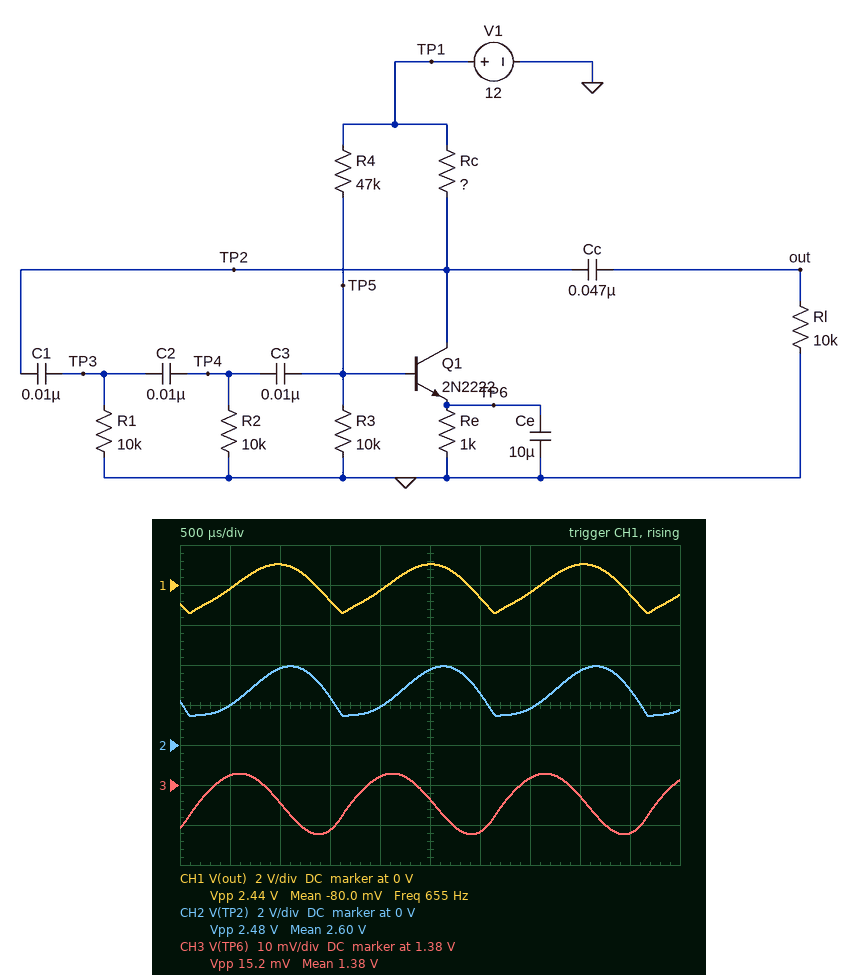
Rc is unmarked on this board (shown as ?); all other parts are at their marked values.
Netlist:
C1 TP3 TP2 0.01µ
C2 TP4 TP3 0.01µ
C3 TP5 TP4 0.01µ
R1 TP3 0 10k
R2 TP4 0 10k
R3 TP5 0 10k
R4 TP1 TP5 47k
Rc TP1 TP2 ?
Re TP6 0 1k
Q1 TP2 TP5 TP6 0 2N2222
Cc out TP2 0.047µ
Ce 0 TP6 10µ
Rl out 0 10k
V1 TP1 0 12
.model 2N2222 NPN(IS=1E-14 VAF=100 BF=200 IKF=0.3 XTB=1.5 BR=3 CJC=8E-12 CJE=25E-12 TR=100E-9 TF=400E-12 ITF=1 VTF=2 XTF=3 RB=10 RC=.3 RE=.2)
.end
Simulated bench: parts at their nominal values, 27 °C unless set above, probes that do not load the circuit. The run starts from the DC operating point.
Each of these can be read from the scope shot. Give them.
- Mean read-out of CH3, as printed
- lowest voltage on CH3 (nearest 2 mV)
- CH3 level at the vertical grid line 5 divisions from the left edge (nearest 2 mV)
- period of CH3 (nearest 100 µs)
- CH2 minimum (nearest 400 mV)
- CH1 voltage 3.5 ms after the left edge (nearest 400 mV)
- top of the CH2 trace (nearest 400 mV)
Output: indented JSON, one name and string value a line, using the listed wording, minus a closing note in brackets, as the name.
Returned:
{
  "Mean read-out of CH3, as printed": "1.38 V",
  "lowest voltage on CH3": "1.368 V",
  "CH3 level at the vertical grid line 5 divisions from the left edge": "1.376 V",
  "period of CH3": "1.5 ms",
  "CH2 minimum": "1.6 V",
  "CH1 voltage 3.5 ms after the left edge": "-400 mV",
  "top of the CH2 trace": "4.0 V"
}
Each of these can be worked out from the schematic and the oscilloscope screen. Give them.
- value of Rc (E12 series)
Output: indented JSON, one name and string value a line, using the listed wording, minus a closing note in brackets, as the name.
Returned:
{
  "value of Rc": "6.8 kΩ"
}
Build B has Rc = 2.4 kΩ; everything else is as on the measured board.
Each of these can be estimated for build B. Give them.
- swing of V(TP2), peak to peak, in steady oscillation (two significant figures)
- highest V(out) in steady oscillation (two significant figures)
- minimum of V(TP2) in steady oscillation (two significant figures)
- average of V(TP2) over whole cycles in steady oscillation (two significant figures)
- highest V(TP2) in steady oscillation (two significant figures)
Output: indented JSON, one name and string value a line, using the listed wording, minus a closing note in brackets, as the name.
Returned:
{
  "swing of V(TP2), peak to peak, in steady oscillation": "5.6 V",
  "highest V(out) in steady oscillation": "2.9 V",
  "minimum of V(TP2) in steady oscillation": "5.7 V",
  "average of V(TP2) over whole cycles in steady oscillation": "8.6 V",
  "highest V(TP2) in steady oscillation": "11 V"
}
